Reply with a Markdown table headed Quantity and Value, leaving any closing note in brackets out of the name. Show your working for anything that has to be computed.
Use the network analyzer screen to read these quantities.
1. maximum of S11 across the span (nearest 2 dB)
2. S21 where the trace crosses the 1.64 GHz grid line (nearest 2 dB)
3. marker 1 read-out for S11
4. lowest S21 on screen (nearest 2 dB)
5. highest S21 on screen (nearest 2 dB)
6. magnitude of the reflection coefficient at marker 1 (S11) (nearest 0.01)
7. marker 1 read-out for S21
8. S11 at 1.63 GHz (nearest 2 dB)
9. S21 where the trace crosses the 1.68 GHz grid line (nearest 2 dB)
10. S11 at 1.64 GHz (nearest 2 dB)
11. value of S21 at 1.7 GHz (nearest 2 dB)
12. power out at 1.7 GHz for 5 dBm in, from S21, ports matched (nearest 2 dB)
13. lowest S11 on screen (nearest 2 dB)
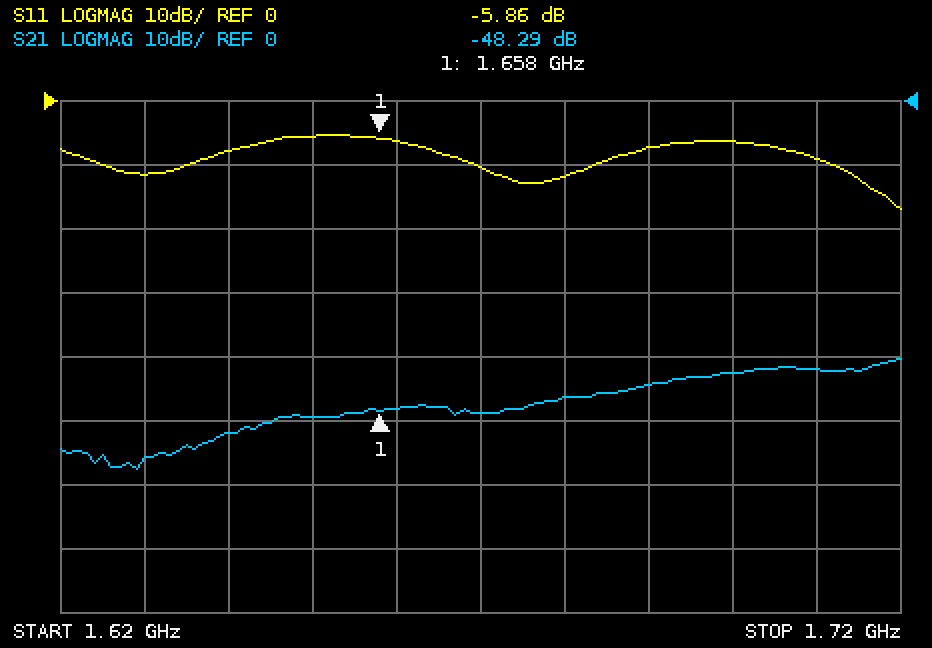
| Quantity | Value |
|---|---|
| maximum of S11 across the span | -6 dB |
| S21 where the trace crosses the 1.64 GHz grid line | -52 dB |
| marker 1 read-out for S11 | -5.86 dB |
| lowest S21 on screen | -58 dB |
| highest S21 on screen | -40 dB |
| magnitude of the reflection coefficient at marker 1 (S11) | 10^(-5.86/20) ≈ 0.51 |
| marker 1 read-out for S21 | -48.29 dB |
| S11 at 1.63 GHz | -12 dB |
| S21 where the trace crosses the 1.68 GHz grid line | -46 dB |
| S11 at 1.64 GHz | -8 dB |
| value of S21 at 1.7 GHz | -42 dB |
| power out at 1.7 GHz for 5 dBm in, from S21, ports matched | 5 dBm + (-42 dB) = -38 dBm |
| lowest S11 on screen | -16 dB |
